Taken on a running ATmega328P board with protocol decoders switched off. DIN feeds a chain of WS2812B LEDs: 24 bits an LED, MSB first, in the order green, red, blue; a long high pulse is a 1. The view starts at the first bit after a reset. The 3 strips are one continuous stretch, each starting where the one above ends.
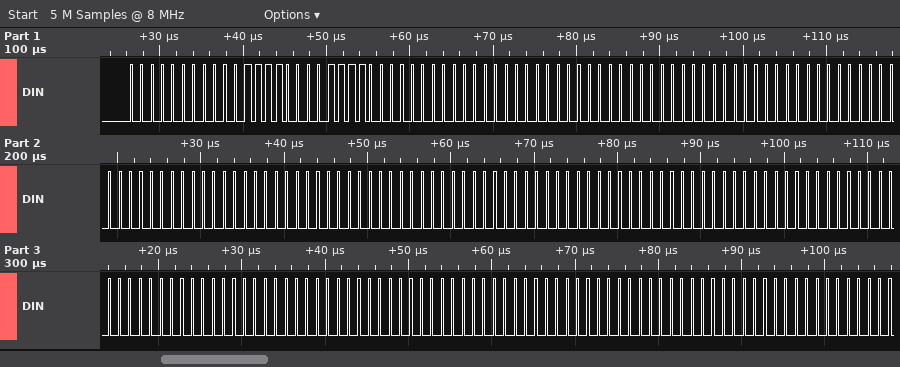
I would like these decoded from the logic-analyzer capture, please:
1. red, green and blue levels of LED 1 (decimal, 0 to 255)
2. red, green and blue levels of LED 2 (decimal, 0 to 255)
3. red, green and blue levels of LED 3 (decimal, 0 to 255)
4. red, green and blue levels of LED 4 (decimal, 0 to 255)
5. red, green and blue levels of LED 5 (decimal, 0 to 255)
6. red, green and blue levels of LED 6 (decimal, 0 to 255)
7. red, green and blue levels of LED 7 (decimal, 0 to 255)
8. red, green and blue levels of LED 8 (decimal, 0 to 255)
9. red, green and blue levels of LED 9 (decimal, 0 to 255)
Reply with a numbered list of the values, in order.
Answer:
1. 30, 0, 30
2. 0, 0, 0
3. 0, 0, 0
4. 0, 0, 0
5. 0, 0, 0
6. 0, 0, 0
7. 0, 0, 0
8. 0, 0, 0
9. 0, 0, 0
